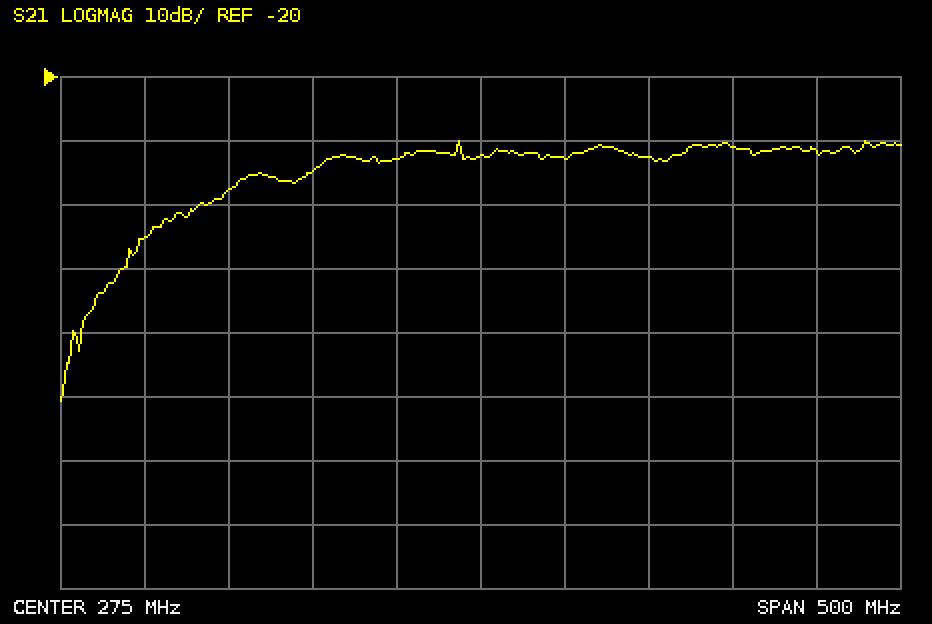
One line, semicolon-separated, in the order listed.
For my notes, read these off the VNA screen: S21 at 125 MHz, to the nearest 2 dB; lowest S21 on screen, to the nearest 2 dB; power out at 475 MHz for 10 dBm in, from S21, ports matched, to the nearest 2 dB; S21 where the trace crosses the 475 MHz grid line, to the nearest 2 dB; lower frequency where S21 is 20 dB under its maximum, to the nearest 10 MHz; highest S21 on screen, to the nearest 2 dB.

-38 dB; -70 dB; -22 dBm; -32 dB; 60 MHz; -30 dB
